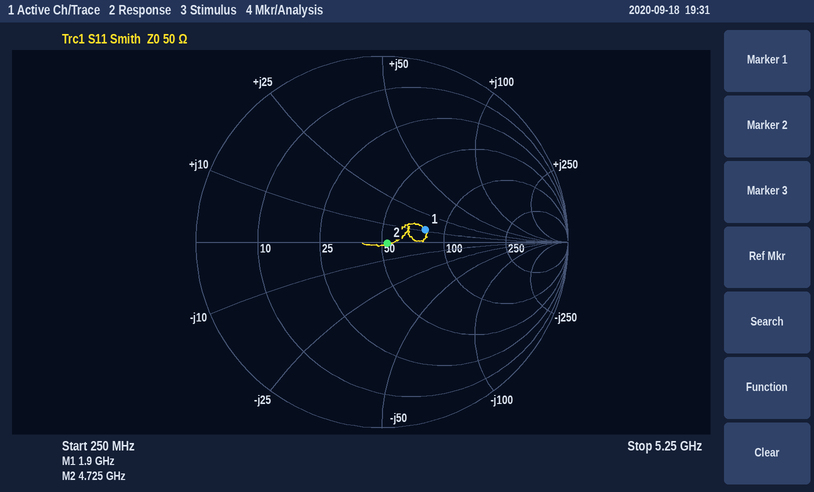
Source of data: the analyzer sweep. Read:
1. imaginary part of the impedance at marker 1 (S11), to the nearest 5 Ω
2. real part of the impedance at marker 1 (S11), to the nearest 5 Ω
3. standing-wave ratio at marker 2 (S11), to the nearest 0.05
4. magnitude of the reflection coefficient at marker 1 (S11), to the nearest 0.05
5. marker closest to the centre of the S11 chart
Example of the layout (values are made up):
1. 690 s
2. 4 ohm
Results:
1. +10 Ω
2. 80 Ω
3. 1.05
4. 0.25
5. marker 2
